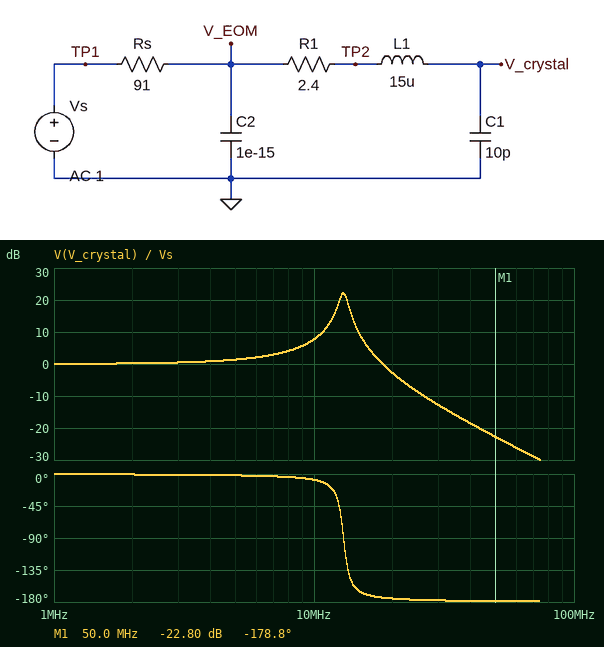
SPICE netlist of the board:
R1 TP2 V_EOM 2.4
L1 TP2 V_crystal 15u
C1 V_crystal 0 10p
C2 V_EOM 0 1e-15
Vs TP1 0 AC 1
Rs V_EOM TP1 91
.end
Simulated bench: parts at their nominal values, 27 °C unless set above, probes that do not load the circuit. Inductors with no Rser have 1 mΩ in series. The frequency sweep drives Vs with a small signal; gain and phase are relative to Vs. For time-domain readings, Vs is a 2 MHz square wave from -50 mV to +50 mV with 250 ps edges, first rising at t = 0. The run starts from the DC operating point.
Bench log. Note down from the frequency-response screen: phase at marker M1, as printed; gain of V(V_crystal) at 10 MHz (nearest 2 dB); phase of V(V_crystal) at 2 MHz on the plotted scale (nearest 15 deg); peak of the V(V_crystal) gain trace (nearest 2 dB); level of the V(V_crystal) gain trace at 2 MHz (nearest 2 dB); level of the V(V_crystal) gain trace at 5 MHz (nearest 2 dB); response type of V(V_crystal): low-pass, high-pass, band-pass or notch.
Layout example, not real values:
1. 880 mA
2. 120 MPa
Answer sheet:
1. -178.8 deg
2. 8 dB
3. 0 deg
4. 22 dB
5. 0 dB
6. 2 dB
7. low-pass
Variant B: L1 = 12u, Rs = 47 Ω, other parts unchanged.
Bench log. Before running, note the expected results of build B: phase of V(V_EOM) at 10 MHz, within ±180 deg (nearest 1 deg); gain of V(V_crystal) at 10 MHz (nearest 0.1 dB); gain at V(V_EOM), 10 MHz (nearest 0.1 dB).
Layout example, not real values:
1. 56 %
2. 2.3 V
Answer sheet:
1. -3 deg
2. 5.6 dB
3. 0 dB
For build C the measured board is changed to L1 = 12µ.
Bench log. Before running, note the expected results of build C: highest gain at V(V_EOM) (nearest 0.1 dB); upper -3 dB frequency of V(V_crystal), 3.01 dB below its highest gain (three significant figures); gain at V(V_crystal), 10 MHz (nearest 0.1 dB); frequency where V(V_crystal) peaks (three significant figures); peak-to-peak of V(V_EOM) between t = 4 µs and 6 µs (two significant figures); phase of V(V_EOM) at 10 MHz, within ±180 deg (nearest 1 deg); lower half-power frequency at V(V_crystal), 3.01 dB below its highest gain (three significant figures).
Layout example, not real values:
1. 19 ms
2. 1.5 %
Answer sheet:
1. 0 dB
2. 15.1 MHz
3. 5.5 dB
4. 14.5 MHz
5. 120 mV
6. -6 deg
7. 13.9 MHz
